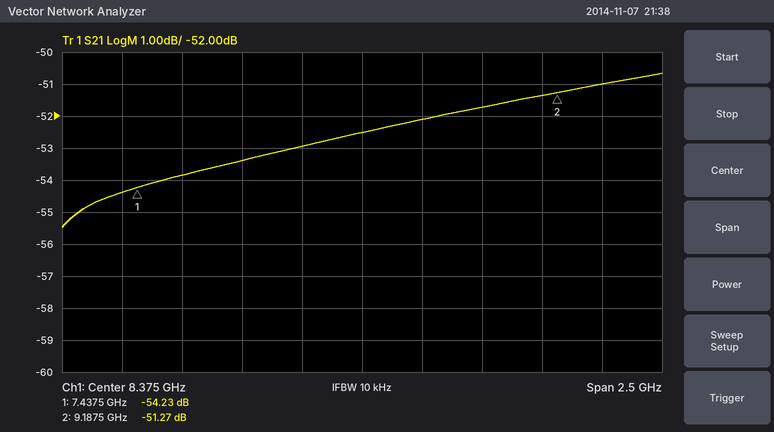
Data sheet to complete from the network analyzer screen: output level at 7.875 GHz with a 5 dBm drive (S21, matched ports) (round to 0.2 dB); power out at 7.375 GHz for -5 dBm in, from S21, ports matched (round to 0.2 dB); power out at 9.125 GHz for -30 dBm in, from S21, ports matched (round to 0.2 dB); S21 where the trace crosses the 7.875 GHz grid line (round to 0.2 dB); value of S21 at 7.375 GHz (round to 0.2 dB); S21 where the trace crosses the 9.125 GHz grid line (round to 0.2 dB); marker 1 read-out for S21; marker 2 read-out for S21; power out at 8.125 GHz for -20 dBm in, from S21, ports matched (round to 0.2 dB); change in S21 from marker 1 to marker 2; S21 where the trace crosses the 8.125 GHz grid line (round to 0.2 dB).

-48.4 dBm
-59.4 dBm
-81.4 dBm
-53.4 dB
-54.4 dB
-51.4 dB
-54.23 dB
-51.27 dB
-73.0 dBm
2.96 dB
-53.0 dB
